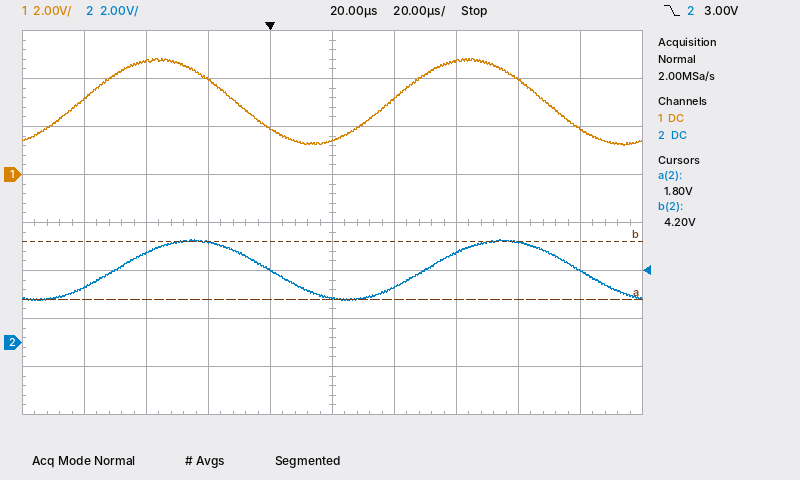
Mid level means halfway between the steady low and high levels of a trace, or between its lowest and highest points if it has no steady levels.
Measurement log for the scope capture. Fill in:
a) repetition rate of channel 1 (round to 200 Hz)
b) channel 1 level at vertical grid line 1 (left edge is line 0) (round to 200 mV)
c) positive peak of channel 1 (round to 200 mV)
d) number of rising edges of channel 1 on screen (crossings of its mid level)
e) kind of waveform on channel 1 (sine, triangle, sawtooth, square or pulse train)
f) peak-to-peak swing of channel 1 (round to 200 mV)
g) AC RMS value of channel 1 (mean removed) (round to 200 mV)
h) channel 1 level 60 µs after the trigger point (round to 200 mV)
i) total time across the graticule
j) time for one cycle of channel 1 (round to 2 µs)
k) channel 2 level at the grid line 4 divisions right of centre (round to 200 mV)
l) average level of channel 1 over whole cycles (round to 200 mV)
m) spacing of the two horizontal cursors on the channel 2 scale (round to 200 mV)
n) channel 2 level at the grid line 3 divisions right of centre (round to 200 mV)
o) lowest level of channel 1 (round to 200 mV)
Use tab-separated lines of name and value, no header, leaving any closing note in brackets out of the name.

repetition rate of channel 1	10.0 kHz
channel 1 level at vertical grid line 1 (left edge is line 0)	3.2 V
positive peak of channel 1	4.8 V
number of rising edges of channel 1 on screen	2
kind of waveform on channel 1	sine
peak-to-peak swing of channel 1	3.6 V
AC RMS value of channel 1 (mean removed)	1.2 V
channel 1 level 60 µs after the trigger point	4.8 V
total time across the graticule	200 µs
time for one cycle of channel 1	100 µs
channel 2 level at the grid line 4 divisions right of centre	3.0 V
average level of channel 1 over whole cycles	3.0 V
spacing of the two horizontal cursors on the channel 2 scale	2.4 V
channel 2 level at the grid line 3 divisions right of centre	4.2 V
lowest level of channel 1	1.2 V
